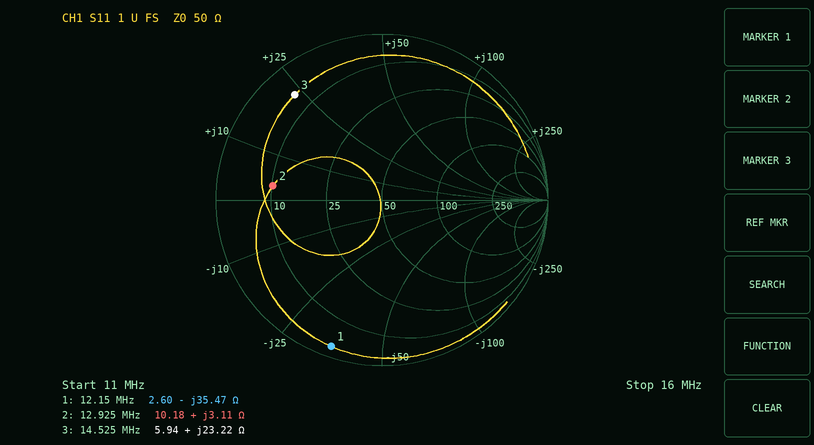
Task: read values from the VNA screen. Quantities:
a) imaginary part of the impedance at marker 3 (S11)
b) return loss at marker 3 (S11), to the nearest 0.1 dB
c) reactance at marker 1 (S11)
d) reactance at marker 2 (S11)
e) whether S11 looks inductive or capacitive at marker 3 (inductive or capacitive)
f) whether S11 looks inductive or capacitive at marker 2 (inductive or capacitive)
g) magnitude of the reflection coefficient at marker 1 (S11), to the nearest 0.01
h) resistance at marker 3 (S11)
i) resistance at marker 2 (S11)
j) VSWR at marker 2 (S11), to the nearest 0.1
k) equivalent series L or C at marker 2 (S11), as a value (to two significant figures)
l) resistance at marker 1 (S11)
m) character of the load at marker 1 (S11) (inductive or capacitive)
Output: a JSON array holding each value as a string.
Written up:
["+23.22 Ω", "1.7 dB", "-35.47 Ω", "+3.11 Ω", "inductive", "inductive", "0.93", "5.94 Ω", "10.18 Ω", "4.9", "38 nH", "2.60 Ω", "capacitive"]
